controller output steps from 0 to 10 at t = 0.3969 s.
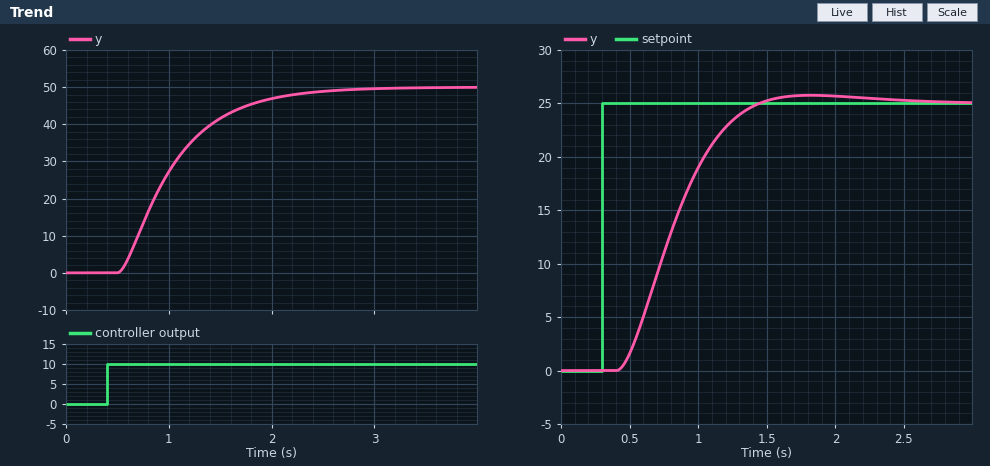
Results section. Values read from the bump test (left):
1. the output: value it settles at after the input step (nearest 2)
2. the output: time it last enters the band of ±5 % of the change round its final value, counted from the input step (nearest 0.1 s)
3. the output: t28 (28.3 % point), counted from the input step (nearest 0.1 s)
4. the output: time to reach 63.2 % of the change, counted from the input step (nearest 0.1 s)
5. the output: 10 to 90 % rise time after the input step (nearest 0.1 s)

50
1.7 s
0.4 s
0.7 s
1.1 s
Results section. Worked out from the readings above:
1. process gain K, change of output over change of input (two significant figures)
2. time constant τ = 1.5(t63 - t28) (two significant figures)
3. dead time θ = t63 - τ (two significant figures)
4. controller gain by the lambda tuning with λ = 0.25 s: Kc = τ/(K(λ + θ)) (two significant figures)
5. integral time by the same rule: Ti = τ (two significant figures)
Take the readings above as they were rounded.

5.0
0.45 s
0.25 s
0.18
0.45 s
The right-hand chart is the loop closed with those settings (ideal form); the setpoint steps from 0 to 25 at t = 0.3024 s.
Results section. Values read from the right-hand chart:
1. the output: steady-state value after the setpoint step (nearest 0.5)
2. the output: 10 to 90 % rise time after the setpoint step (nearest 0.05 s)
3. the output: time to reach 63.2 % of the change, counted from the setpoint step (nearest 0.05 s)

25.0
0.65 s
0.60 s
